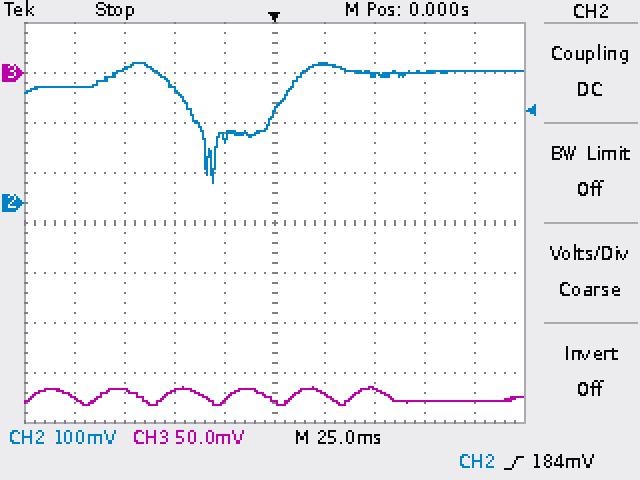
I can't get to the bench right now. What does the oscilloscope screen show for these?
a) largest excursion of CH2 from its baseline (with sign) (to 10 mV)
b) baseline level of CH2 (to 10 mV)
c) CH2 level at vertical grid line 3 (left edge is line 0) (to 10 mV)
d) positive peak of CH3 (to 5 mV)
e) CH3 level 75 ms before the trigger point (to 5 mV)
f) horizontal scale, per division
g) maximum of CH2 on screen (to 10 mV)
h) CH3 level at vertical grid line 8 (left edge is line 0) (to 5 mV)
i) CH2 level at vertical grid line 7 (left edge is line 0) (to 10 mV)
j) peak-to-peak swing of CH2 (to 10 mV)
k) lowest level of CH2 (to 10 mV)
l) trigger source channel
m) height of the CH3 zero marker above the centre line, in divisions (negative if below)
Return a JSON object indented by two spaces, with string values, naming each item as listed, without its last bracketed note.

{
  "largest excursion of CH2 from its baseline (with sign)": "-220 mV",
  "baseline level of CH2": "260 mV",
  "CH2 level at vertical grid line 3 (left edge is line 0)": "230 mV",
  "positive peak of CH3": "-315 mV",
  "CH3 level 75 ms before the trigger point": "-315 mV",
  "horizontal scale, per division": "25 ms",
  "maximum of CH2 on screen": "280 mV",
  "CH3 level at vertical grid line 8 (left edge is line 0)": "-330 mV",
  "CH2 level at vertical grid line 7 (left edge is line 0)": "260 mV",
  "peak-to-peak swing of CH2": "240 mV",
  "lowest level of CH2": "40 mV",
  "trigger source channel": "CH2",
  "height of the CH3 zero marker above the centre line, in divisions": "+3.0 div"
}
